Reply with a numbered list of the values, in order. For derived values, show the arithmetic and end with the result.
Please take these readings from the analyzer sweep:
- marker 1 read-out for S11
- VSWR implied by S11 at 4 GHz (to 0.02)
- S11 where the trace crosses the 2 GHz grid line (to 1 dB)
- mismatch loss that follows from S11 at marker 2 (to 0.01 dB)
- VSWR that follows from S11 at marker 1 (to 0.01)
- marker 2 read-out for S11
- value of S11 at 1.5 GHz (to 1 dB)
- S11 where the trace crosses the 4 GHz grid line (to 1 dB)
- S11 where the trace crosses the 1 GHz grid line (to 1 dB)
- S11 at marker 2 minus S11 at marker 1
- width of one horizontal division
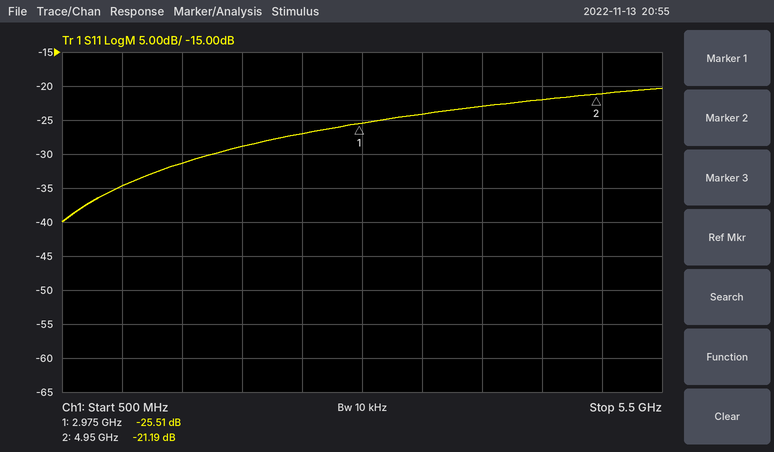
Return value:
1. -25.51 dB
2. |Γ| = 10^(-23/20) = 0.0708; VSWR = (1 + 0.0708)/(1 − 0.0708) ≈ 1.15, so 1.16 to the nearest 0.02
3. -29 dB
4. −10 log10(1 − 10^(-21.19/10)) ≈ 0.03 dB
5. (1 + 0.0530)/(1 − 0.0530) ≈ 1.11
6. -21.19 dB
7. -31 dB
8. -23 dB
9. -35 dB
10. -21.19 − (-25.51) = 4.32 dB
11. 500 MHz
